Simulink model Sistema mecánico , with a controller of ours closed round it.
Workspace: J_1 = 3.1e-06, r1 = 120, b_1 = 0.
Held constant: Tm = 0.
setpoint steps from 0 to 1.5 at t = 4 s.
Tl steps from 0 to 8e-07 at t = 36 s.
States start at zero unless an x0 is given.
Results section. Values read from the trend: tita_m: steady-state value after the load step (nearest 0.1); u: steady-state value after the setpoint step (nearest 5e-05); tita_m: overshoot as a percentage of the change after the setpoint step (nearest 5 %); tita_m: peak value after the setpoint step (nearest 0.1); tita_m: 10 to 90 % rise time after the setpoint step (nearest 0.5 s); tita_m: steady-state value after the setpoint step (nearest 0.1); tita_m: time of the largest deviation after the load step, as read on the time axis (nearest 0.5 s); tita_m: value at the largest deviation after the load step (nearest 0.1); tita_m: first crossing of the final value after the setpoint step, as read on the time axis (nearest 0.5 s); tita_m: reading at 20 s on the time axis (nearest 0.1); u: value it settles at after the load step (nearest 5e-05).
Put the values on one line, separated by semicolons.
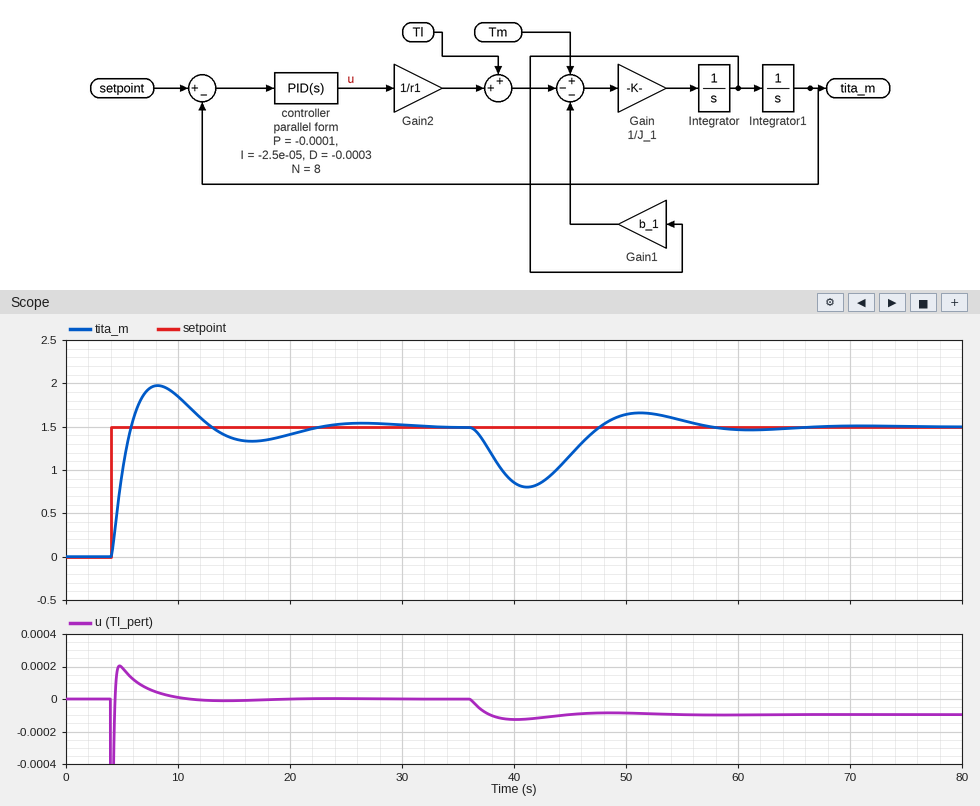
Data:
1.5; 0.00000; 30 %; 2.0; 1.5 s; 1.5; 41.0 s; 0.8; 6.0 s; 1.4; -0.00010
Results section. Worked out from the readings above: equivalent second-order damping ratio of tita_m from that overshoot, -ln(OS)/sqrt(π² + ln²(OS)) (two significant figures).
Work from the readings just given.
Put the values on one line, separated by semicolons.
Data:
0.36
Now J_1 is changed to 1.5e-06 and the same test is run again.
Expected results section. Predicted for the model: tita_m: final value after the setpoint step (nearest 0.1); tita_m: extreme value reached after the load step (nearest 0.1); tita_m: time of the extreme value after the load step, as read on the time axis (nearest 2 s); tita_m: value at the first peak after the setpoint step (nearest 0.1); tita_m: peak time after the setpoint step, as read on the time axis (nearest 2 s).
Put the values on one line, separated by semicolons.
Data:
1.5; 0.9; 40 s; 1.8; 6 s
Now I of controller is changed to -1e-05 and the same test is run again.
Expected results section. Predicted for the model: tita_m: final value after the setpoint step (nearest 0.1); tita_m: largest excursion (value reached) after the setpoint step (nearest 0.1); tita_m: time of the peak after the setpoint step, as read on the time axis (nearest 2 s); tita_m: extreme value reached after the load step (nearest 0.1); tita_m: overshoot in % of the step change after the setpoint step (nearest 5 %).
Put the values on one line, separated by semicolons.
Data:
1.5; 1.9; 8 s; 0.7; 25 %
